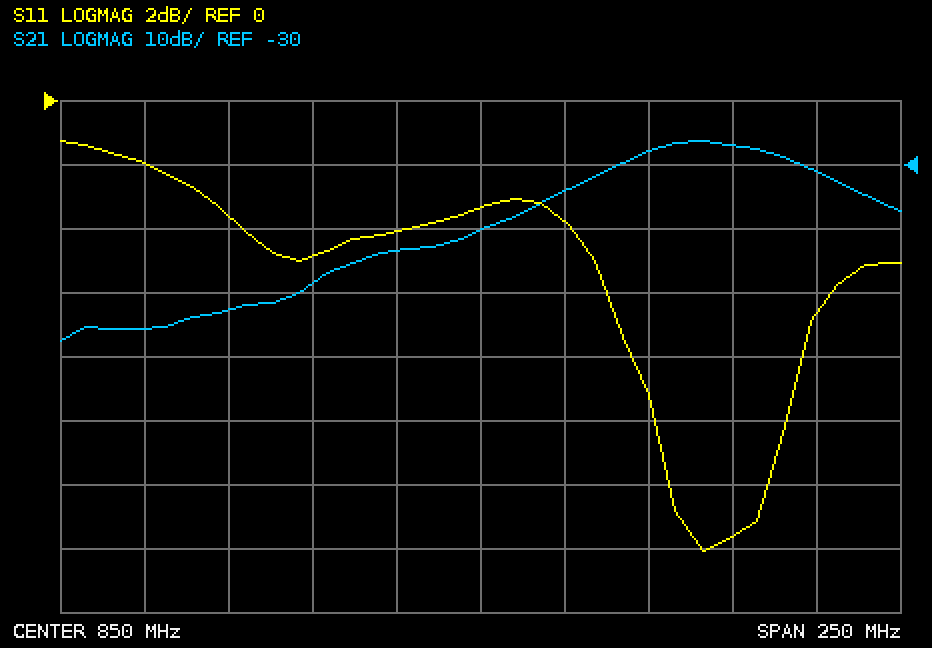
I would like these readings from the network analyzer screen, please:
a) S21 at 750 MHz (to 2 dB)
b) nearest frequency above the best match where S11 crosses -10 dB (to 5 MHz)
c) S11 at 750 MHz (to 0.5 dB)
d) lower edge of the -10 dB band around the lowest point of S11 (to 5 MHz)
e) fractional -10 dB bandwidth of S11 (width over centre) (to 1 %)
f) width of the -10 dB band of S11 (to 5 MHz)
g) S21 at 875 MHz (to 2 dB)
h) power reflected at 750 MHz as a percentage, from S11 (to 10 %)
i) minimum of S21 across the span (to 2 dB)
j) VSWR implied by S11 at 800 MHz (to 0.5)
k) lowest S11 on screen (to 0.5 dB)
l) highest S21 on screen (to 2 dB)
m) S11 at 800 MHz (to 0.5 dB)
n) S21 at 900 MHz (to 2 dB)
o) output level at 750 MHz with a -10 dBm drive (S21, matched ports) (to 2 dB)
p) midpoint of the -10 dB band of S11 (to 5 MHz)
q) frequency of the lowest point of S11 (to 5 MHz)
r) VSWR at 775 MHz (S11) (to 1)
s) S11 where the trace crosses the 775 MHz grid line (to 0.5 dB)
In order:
-56 dB
940 MHz
-2.0 dB
900 MHz
4 %
40 MHz
-34 dB
60 %
-58 dB
3.5
-14.0 dB
-26 dB
-5.0 dB
-28 dB
-66 dBm
920 MHz
915 MHz
5
-3.5 dB
